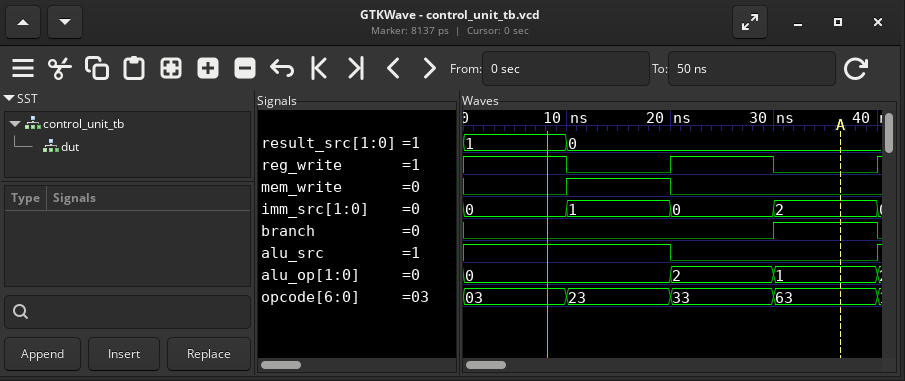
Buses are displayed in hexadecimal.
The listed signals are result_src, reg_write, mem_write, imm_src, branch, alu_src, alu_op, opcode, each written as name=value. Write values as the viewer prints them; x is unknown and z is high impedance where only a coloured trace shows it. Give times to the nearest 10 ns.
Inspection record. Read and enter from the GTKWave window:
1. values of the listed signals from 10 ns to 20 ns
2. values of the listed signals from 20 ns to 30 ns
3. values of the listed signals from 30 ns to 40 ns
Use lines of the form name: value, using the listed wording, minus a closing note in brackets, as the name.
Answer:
values of the listed signals from 10 ns to 20 ns: result_src=0, reg_write=0, mem_write=1, imm_src=1, branch=0, alu_src=1, alu_op=0, opcode=23
values of the listed signals from 20 ns to 30 ns: result_src=0, reg_write=1, mem_write=0, imm_src=0, branch=0, alu_src=0, alu_op=2, opcode=33
values of the listed signals from 30 ns to 40 ns: result_src=0, reg_write=0, mem_write=0, imm_src=2, branch=1, alu_src=0, alu_op=1, opcode=63
